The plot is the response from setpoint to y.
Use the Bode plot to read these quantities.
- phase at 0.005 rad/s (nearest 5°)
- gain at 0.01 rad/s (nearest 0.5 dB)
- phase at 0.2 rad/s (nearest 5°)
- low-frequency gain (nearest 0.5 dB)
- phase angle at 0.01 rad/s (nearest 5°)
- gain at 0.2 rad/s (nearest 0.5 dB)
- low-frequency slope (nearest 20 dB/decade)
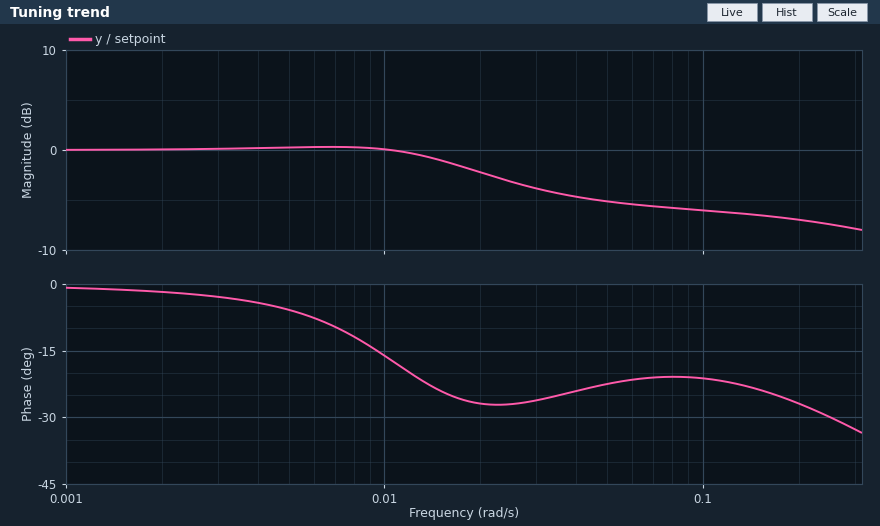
-5°
0.0 dB
-25°
0.0 dB
-15°
-7.0 dB
0 dB/decade
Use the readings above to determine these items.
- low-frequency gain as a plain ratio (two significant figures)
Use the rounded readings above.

1.0
